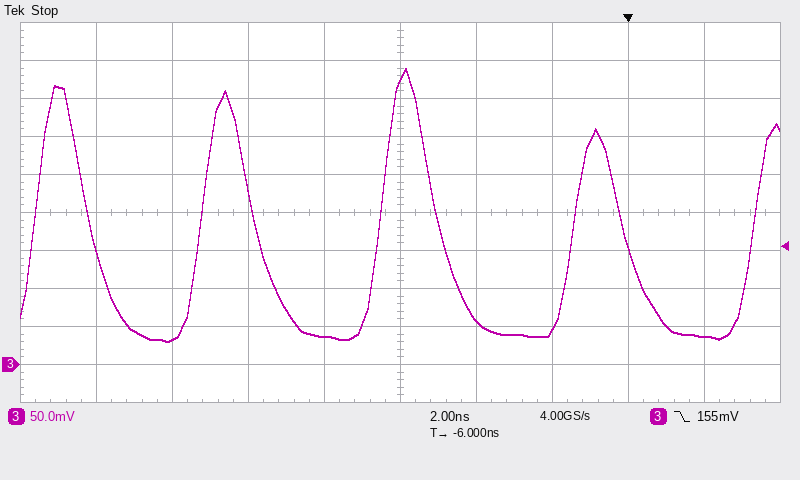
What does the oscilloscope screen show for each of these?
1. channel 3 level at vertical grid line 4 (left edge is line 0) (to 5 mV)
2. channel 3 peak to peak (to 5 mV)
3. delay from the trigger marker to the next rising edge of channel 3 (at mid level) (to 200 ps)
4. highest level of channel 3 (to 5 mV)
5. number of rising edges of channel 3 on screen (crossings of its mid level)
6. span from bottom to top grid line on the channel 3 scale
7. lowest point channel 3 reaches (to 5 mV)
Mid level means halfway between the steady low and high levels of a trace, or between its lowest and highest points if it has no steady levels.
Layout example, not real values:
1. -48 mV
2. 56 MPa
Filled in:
1. 35 mV
2. 360 mV
3. 3.4 ns
4. 390 mV
5. 5
6. 500 mV
7. 30 mV
